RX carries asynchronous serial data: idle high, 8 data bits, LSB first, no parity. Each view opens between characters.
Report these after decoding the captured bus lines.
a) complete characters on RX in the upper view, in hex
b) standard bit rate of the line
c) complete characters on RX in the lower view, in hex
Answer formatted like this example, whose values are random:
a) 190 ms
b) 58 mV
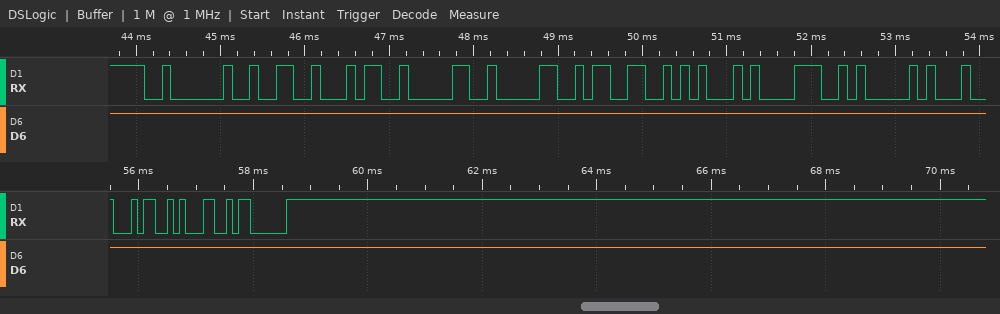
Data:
a) 02, 32, 34, 30, 30, 33, 45, 38, 41
b) 9600 baud
c) 34, 31, 03
